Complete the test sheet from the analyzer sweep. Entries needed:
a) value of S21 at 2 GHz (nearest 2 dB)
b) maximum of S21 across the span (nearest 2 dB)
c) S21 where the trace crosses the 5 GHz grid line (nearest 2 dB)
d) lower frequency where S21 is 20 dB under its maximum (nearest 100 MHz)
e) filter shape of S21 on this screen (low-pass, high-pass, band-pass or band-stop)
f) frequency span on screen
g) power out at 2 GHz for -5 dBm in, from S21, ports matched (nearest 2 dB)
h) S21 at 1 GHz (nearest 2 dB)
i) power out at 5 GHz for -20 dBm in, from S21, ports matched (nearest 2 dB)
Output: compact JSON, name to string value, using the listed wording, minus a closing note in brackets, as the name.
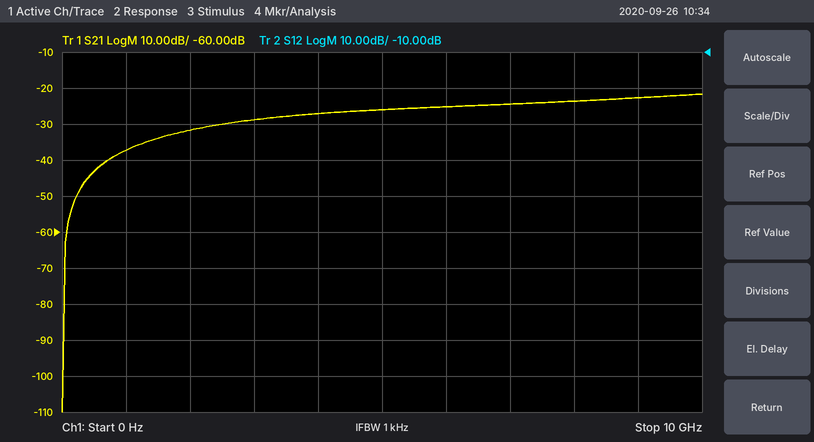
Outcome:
{"value of S21 at 2 GHz": "-32 dB", "maximum of S21 across the span": "-22 dB", "S21 where the trace crosses the 5 GHz grid line": "-26 dB", "lower frequency where S21 is 20 dB under its maximum": "600 MHz", "filter shape of S21 on this screen": "high-pass", "frequency span on screen": "10 GHz", "power out at 2 GHz for -5 dBm in, from S21, ports matched": "-36 dBm", "S21 at 1 GHz": "-38 dB", "power out at 5 GHz for -20 dBm in, from S21, ports matched": "-46 dBm"}
